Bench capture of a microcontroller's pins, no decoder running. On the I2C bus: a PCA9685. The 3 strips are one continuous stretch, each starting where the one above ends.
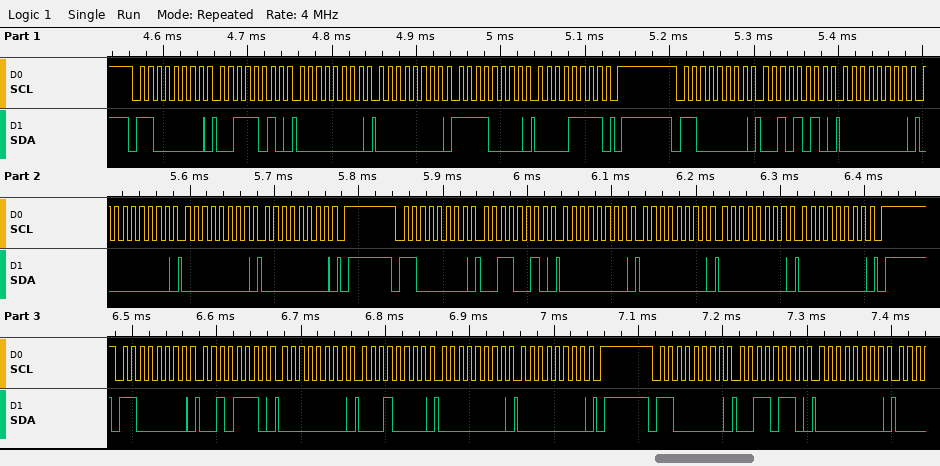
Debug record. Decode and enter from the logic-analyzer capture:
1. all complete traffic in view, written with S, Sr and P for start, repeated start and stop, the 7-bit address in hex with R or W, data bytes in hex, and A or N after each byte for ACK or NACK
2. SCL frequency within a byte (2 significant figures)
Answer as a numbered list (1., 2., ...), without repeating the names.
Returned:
1. S 60W A 3A A 00 A 00 A F0 A 0F A P S 60W A 2A A 00 A 00 A 00 A 00 A P S 60W A 32 A 00 A 00 A 00 A 00 A P S 60W A 2E A 00 A 10 A 00 A 00 A P S 60W A 36 A 00 A
2. 100 kHz
